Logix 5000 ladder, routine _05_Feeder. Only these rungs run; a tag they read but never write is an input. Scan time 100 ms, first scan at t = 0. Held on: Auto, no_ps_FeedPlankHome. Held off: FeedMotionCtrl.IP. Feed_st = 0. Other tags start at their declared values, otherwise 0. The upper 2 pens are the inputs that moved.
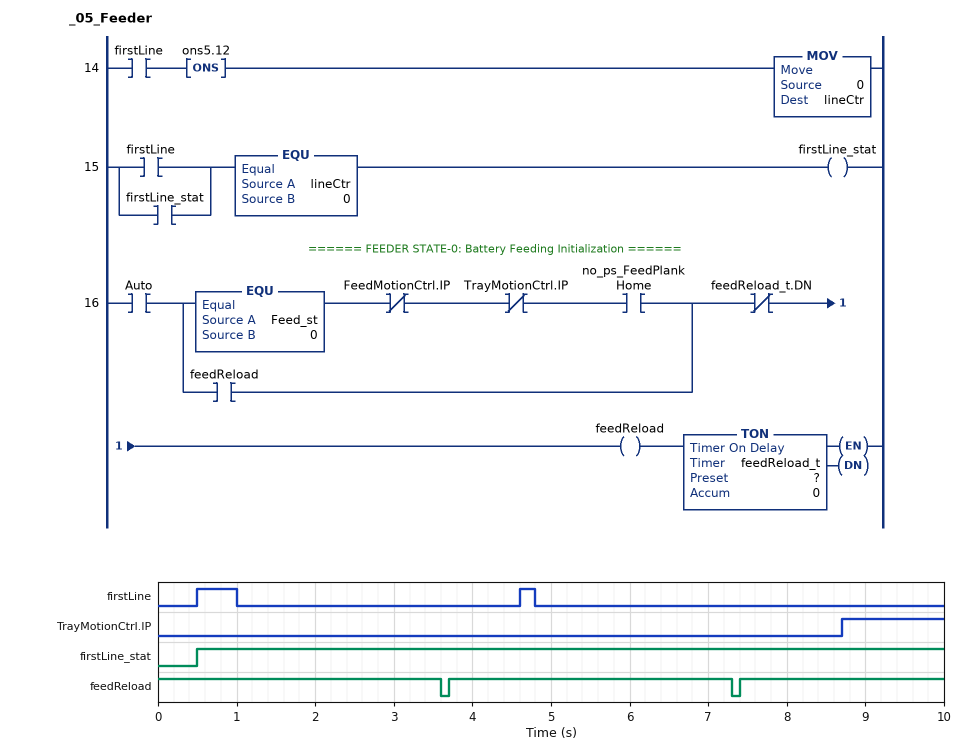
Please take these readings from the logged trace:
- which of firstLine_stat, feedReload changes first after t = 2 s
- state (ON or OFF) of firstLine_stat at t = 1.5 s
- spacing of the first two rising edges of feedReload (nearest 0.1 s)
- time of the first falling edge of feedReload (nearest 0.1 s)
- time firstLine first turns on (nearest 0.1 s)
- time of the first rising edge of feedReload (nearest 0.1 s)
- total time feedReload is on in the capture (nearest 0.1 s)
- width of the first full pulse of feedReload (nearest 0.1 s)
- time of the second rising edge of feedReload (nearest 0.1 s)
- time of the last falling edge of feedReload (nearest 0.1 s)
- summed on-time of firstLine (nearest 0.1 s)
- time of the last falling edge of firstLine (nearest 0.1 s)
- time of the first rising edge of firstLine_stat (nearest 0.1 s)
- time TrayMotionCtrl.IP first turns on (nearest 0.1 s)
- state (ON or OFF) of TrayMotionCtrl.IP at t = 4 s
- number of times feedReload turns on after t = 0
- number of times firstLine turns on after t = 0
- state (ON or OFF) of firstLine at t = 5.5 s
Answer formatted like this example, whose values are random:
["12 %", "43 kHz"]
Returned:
["feedReload", "ON", "3.7 s", "3.6 s", "0.5 s", "3.7 s", "9.8 s", "3.6 s", "7.4 s", "7.3 s", "0.7 s", "4.8 s", "0.5 s", "8.7 s", "OFF", "2", "2", "OFF"]
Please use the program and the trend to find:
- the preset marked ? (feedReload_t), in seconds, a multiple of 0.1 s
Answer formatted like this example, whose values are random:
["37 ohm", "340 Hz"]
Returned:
["3.5 s"]
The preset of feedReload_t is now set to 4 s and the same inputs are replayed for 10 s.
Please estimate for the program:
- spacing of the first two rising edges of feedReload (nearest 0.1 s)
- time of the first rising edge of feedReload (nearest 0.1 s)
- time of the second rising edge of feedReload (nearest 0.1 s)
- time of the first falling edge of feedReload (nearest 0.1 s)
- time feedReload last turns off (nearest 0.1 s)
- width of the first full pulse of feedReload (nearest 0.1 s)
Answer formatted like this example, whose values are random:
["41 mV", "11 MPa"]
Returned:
["4.2 s", "4.2 s", "8.4 s", "4.1 s", "8.3 s", "4.1 s"]
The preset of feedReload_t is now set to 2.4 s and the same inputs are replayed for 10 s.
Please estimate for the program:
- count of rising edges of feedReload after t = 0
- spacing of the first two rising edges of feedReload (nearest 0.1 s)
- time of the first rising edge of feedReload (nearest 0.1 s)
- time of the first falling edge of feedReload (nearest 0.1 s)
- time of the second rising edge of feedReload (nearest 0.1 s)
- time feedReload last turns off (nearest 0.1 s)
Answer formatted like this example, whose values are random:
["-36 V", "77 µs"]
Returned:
["3", "2.6 s", "2.6 s", "2.5 s", "5.2 s", "7.7 s"]
